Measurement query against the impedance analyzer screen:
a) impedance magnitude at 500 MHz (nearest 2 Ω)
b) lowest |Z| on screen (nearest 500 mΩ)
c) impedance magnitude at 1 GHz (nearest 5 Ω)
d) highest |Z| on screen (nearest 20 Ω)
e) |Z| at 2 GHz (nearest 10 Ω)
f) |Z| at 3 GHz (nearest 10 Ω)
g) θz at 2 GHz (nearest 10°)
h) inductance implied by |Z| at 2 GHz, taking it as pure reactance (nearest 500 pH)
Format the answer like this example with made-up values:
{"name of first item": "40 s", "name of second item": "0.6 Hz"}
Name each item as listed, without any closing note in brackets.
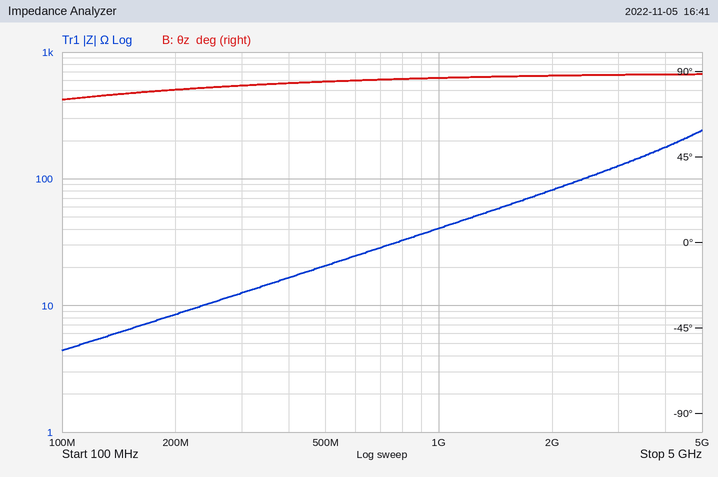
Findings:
{"impedance magnitude at 500 MHz": "20 Ω", "lowest |Z| on screen": "4.5 Ω", "impedance magnitude at 1 GHz": "40 Ω", "highest |Z| on screen": "240 Ω", "|Z| at 2 GHz": "80 Ω", "|Z| at 3 GHz": "130 Ω", "θz at 2 GHz": "90°", "inductance implied by |Z| at 2 GHz, taking it as pure reactance": "6.5 nH"}
